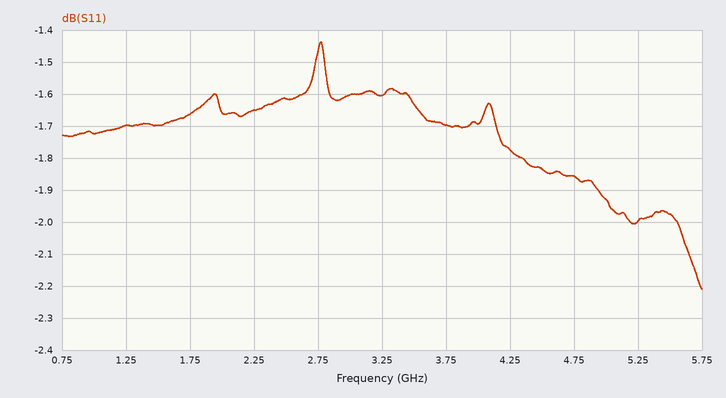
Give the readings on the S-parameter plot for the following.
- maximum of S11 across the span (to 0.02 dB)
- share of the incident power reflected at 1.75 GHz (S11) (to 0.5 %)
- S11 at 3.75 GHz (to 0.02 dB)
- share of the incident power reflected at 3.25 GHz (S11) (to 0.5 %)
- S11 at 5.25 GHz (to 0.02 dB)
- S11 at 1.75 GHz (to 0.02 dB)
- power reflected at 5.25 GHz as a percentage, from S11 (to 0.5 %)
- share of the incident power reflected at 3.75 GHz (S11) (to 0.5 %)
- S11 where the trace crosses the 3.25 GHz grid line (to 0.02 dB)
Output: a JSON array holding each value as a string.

["-1.44 dB", "68.0 %", "-1.70 dB", "69.0 %", "-2.00 dB", "-1.66 dB", "63.0 %", "67.5 %", "-1.60 dB"]
